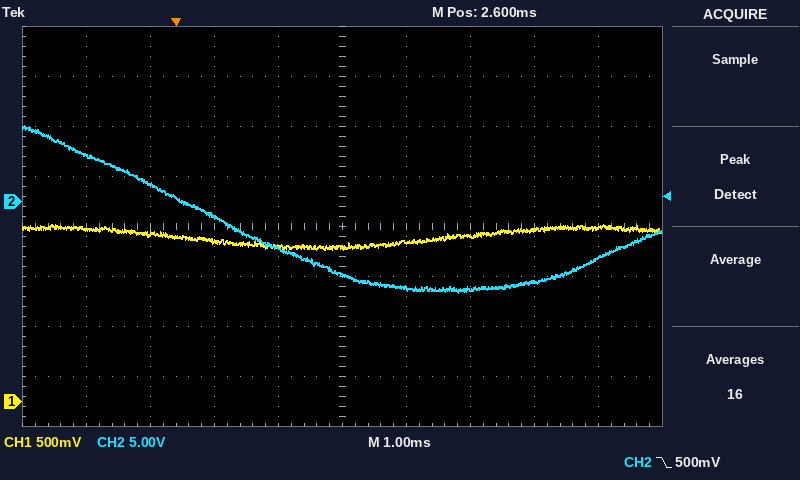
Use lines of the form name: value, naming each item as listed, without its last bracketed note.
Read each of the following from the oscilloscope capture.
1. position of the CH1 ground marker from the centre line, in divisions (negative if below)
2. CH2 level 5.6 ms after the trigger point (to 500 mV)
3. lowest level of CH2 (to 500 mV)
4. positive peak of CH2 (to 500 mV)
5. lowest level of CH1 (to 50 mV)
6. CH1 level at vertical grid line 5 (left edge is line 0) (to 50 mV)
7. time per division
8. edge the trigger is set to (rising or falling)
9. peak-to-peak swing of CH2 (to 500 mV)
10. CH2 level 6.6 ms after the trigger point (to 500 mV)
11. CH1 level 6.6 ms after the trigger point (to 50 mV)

position of the CH1 ground marker from the centre line, in divisions: -3.5 div
CH2 level 5.6 ms after the trigger point: -8.0 V
lowest level of CH2: -9.0 V
positive peak of CH2: 7.5 V
lowest level of CH1: 1.50 V
CH1 level at vertical grid line 5 (left edge is line 0): 1.55 V
time per division: 1 ms
edge the trigger is set to: falling
peak-to-peak swing of CH2: 16.5 V
CH2 level 6.6 ms after the trigger point: -5.5 V
CH1 level 6.6 ms after the trigger point: 1.75 V
